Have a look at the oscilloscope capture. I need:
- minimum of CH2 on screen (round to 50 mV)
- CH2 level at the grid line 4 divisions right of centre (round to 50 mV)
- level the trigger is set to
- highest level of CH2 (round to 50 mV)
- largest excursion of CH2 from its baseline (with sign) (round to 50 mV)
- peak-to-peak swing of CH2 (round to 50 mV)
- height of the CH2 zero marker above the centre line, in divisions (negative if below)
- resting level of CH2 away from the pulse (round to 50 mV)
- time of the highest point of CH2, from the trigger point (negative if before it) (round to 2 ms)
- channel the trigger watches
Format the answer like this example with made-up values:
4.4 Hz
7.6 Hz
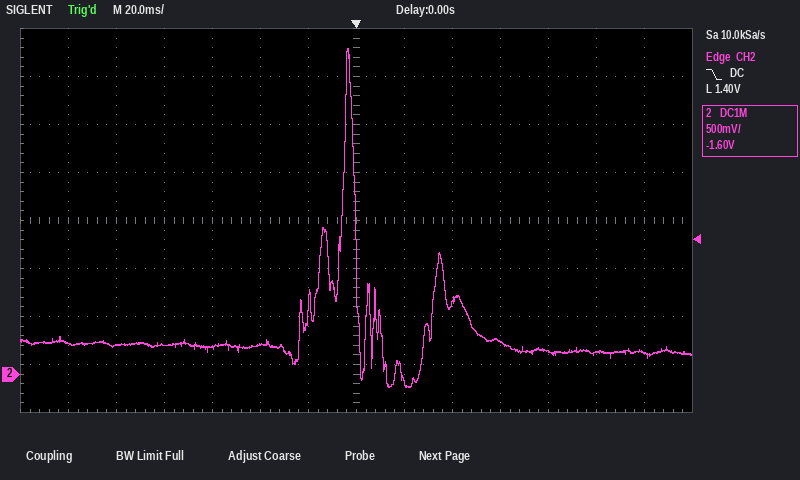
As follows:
-150 mV
250 mV
1.40 V
3.40 V
+3.10 V
3.55 V
-3.2 div
300 mV
-4 ms
CH2
